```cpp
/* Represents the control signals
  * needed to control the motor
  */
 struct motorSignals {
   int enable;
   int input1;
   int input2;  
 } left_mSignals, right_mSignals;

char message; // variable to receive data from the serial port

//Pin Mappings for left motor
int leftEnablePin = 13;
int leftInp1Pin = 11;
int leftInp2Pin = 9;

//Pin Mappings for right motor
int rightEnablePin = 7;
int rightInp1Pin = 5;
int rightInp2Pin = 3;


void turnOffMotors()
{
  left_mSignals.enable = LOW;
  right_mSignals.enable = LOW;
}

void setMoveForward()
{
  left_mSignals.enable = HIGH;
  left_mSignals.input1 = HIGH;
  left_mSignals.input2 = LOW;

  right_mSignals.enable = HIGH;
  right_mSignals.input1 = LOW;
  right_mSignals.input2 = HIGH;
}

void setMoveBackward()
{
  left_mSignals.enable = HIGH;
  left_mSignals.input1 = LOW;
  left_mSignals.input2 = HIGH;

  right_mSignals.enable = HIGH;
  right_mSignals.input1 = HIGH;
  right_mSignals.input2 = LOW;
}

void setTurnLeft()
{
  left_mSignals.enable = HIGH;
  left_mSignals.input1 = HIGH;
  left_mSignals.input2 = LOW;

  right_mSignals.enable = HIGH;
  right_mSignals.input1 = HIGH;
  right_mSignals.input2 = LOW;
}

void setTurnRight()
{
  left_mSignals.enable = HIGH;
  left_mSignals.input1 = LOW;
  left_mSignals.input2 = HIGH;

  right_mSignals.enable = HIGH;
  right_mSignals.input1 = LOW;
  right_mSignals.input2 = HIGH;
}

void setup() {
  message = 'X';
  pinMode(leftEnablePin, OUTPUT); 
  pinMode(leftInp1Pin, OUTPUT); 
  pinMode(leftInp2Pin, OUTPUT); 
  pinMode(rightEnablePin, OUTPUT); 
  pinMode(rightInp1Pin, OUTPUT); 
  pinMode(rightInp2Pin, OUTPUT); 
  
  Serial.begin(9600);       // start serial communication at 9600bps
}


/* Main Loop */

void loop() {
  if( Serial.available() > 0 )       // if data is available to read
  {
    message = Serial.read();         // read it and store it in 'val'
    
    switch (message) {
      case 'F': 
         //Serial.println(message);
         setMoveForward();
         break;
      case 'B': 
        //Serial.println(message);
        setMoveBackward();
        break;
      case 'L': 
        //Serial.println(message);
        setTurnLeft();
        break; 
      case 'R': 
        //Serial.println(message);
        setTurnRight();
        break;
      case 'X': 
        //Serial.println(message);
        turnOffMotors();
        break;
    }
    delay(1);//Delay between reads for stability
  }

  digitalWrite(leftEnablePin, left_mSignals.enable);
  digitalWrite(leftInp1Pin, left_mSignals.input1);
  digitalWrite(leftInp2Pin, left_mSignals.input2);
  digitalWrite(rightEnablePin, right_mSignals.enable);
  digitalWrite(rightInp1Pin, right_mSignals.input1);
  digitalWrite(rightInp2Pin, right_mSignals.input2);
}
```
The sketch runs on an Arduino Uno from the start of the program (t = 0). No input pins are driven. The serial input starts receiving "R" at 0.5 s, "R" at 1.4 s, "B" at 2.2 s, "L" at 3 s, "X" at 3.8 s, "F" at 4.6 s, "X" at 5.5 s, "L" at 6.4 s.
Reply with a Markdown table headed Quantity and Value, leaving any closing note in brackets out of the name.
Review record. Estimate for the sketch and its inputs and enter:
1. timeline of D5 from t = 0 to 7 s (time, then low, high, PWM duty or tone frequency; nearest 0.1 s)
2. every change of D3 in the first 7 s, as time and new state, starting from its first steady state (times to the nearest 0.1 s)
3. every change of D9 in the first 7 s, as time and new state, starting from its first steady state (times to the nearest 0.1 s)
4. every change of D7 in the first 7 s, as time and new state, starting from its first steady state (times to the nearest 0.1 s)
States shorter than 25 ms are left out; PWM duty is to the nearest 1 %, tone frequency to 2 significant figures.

| Quantity | Value |
|---|---|
| timeline of D5 from t = 0 to 7 s | 0 s low; 2.2 s high; 4.6 s low; 6.4 s high |
| every change of D3 in the first 7 s, as time and new state, starting from its first steady state | 0 s low; 0.5 s high; 2.2 s low; 4.6 s high; 6.4 s low |
| every change of D9 in the first 7 s, as time and new state, starting from its first steady state | 0 s low; 0.5 s high; 3 s low |
| every change of D7 in the first 7 s, as time and new state, starting from its first steady state | 0 s low; 0.5 s high; 3.8 s low; 4.6 s high; 5.5 s low; 6.4 s high |
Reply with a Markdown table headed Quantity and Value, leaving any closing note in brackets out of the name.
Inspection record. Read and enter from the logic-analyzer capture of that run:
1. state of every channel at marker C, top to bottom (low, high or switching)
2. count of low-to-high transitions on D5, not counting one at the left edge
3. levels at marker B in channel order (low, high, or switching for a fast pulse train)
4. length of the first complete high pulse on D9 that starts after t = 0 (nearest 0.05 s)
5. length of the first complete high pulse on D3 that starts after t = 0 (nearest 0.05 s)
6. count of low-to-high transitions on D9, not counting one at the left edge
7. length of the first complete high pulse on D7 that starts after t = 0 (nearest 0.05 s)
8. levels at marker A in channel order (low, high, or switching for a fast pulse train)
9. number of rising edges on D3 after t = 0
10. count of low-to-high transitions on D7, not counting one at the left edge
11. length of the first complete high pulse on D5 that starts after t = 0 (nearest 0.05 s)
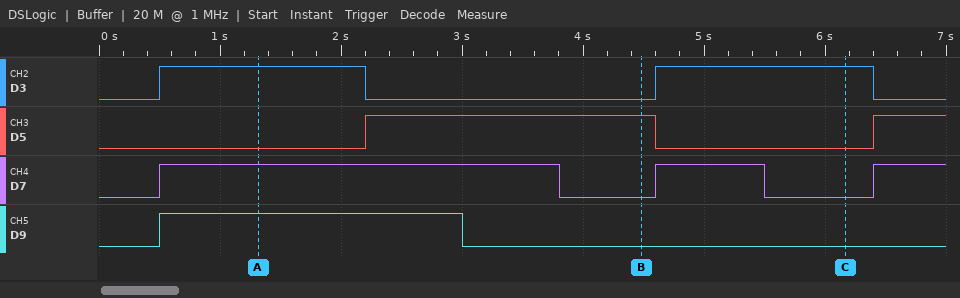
| Quantity | Value |
|---|---|
| state of every channel at marker C, top to bottom | D3 high, D5 low, D7 low, D9 low |
| count of low-to-high transitions on D5, not counting one at the left edge | 2 |
| levels at marker B in channel order | D3 low, D5 high, D7 low, D9 low |
| length of the first complete high pulse on D9 that starts after t = 0 | 2.50 s |
| length of the first complete high pulse on D3 that starts after t = 0 | 1.70 s |
| count of low-to-high transitions on D9, not counting one at the left edge | 1 |
| length of the first complete high pulse on D7 that starts after t = 0 | 3.30 s |
| levels at marker A in channel order | D3 high, D5 low, D7 high, D9 high |
| number of rising edges on D3 after t = 0 | 2 |
| count of low-to-high transitions on D7, not counting one at the left edge | 3 |
| length of the first complete high pulse on D5 that starts after t = 0 | 2.40 s |
